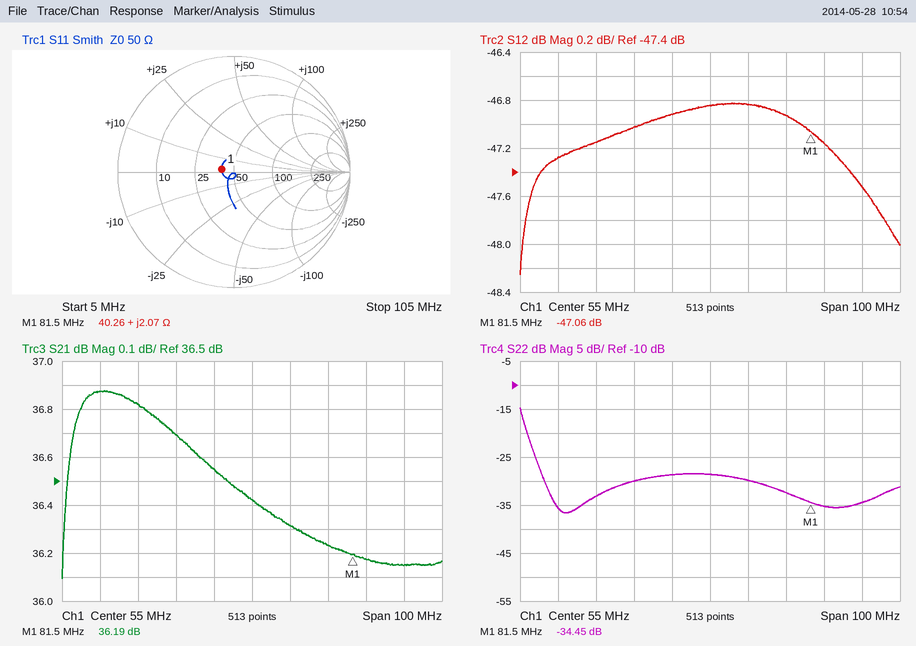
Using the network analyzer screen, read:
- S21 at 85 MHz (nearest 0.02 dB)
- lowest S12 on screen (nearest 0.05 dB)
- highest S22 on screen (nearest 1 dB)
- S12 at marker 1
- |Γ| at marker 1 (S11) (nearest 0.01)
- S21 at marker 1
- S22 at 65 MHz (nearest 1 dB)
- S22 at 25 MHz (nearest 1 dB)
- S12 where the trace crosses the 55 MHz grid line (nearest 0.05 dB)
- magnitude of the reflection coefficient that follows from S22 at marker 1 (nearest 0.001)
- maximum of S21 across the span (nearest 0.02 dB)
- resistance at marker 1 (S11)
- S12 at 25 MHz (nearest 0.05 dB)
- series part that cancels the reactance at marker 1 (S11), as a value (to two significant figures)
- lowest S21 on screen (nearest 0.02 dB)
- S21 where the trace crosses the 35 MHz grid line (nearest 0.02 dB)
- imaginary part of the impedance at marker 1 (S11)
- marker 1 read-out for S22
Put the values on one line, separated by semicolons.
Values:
36.18 dB; -48.25 dB; -15 dB; -47.06 dB; 0.11; 36.19 dB; -30 dB; -33 dB; -46.85 dB; 0.019; 36.88 dB; 40.26 Ω; -47.15 dB; 940 pF; 36.10 dB; 36.70 dB; +2.07 Ω; -34.45 dB
